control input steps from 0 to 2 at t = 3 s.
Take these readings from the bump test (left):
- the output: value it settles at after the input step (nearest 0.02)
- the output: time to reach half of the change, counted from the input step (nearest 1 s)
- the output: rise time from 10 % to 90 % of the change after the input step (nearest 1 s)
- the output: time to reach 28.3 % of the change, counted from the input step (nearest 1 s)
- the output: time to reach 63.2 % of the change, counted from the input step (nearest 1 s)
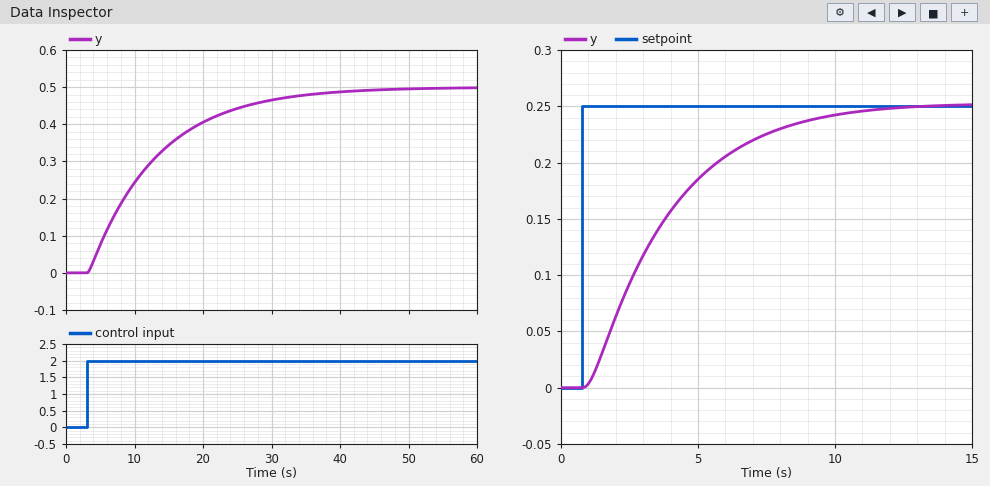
0.50
7 s
22 s
4 s
10 s
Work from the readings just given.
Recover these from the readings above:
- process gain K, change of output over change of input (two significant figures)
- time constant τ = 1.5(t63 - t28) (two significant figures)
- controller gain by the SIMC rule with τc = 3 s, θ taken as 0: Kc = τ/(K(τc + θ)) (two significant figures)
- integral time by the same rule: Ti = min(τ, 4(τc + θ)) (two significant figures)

0.25
9.0 s
12
9.0 s
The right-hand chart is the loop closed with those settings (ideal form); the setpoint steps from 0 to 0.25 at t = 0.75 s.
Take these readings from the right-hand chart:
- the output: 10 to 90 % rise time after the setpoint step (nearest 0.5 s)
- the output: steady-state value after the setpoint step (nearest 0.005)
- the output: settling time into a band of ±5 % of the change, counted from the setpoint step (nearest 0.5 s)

6.0 s
0.250
8.5 s
